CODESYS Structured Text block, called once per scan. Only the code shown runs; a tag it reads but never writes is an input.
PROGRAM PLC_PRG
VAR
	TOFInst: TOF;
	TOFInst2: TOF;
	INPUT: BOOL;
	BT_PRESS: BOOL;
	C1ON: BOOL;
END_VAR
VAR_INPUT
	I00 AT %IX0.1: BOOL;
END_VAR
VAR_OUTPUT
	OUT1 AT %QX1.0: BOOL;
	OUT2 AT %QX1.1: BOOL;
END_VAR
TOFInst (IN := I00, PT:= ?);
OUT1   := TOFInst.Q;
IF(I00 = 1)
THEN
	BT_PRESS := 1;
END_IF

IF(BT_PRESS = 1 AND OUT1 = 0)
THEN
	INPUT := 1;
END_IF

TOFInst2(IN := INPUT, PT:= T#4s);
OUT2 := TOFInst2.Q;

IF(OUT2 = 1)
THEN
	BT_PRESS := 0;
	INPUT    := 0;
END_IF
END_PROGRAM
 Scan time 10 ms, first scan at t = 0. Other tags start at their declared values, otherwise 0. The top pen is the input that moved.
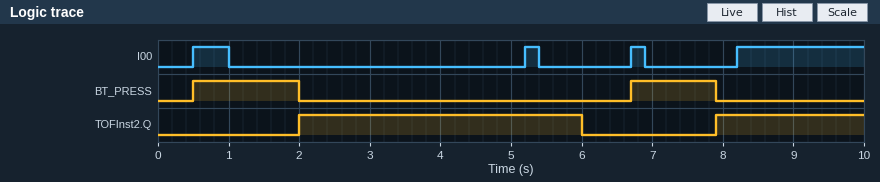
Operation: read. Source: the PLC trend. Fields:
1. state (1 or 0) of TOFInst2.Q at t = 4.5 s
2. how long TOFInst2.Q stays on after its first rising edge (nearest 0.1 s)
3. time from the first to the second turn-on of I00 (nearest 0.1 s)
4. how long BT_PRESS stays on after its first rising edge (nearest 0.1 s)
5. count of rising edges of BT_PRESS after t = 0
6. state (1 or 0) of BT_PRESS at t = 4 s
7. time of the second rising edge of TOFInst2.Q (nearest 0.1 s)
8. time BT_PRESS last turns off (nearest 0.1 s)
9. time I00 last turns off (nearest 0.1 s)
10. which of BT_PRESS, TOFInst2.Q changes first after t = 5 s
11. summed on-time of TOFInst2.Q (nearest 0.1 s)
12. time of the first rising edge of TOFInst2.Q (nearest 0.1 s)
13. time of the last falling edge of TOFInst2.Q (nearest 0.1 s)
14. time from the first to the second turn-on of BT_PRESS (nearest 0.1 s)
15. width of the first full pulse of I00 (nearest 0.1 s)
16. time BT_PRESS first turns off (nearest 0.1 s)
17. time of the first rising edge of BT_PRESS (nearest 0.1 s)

1
4.0 s
4.7 s
1.5 s
2
0
7.9 s
7.9 s
6.9 s
TOFInst2.Q
6.1 s
2.0 s
6.0 s
6.2 s
0.5 s
2.0 s
0.5 s
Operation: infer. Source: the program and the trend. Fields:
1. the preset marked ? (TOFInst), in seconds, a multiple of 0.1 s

1.0 s
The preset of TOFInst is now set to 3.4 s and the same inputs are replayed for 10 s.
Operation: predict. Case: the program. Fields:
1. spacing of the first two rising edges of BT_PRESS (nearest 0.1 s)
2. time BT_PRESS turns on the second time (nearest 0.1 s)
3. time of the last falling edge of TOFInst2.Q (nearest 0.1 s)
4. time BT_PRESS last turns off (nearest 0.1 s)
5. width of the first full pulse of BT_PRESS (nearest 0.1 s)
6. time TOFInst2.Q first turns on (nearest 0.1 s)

7.9 s
8.4 s
8.4 s
4.4 s
3.9 s
4.4 s
